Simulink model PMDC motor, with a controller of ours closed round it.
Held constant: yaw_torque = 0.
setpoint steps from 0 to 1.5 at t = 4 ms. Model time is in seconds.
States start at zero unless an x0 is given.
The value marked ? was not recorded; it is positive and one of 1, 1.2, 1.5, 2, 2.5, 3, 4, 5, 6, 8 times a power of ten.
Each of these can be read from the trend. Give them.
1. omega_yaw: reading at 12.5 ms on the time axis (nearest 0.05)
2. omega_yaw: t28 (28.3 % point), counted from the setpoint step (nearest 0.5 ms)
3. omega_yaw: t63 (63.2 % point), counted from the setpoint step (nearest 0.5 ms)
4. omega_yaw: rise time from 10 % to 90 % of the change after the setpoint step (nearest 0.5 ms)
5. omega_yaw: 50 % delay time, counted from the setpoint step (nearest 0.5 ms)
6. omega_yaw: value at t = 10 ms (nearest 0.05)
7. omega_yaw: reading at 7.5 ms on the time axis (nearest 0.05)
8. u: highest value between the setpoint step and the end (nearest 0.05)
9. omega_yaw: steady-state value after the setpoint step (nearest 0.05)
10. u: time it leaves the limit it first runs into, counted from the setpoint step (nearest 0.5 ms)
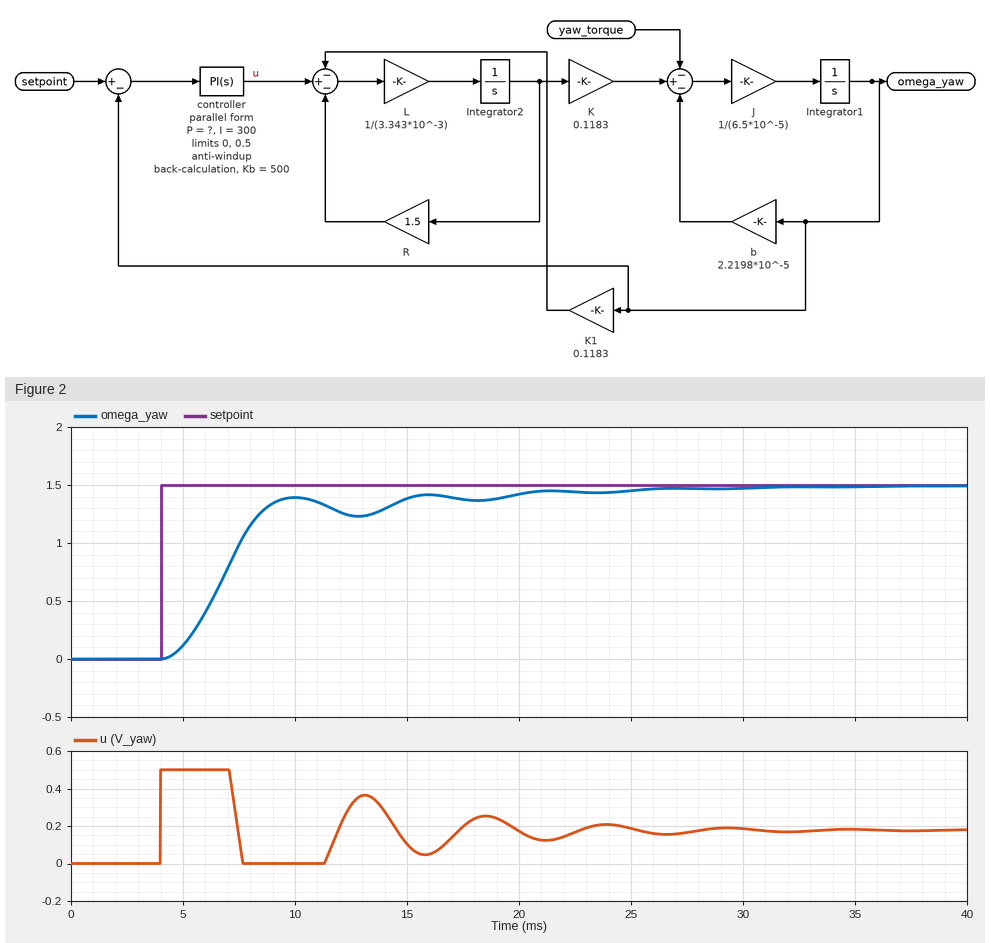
1.25
2.0 ms
3.5 ms
4.0 ms
3.0 ms
1.40
1.00
0.50
1.50
3.0 ms
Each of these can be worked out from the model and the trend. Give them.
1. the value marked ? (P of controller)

2.5
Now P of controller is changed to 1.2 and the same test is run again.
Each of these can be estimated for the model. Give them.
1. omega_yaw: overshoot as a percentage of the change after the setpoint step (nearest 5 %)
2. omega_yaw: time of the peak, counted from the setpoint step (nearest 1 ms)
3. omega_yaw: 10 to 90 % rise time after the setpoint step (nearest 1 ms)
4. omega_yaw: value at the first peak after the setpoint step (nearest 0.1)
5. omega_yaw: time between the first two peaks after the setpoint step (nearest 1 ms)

15 %
7 ms
3 ms
1.7
8 ms
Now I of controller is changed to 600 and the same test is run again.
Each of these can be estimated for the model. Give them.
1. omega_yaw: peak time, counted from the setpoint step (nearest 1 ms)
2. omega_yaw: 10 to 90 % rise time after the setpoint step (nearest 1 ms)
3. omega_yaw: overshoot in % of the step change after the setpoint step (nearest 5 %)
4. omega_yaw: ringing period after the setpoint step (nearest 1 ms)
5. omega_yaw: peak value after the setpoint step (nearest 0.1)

6 ms
3 ms
10 %
6 ms
1.6
